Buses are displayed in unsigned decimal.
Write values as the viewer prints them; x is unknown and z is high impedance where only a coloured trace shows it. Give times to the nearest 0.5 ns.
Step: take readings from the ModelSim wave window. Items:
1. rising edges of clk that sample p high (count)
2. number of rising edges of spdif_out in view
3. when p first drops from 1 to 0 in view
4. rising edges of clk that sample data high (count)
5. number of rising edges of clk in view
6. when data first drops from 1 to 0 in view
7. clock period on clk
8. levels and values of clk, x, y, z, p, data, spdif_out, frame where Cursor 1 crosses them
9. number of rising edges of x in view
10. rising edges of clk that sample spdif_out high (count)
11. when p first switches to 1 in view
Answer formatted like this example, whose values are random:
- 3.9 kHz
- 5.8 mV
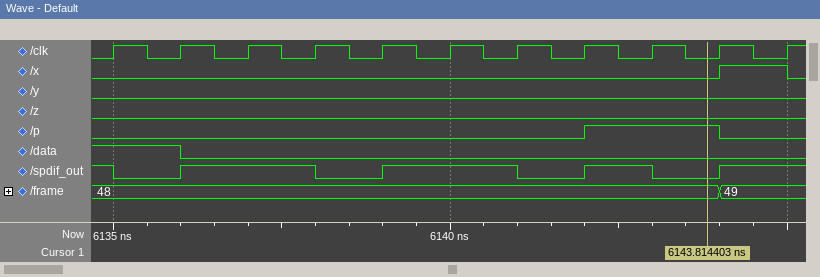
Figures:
- 2
- 4
- 6144 ns
- 2
- 11
- 6136 ns
- 1 ns
- clk=0, x=0, y=0, z=0, p=1, data=0, spdif_out=0, frame=48
- 1
- 7
- 6142 ns
